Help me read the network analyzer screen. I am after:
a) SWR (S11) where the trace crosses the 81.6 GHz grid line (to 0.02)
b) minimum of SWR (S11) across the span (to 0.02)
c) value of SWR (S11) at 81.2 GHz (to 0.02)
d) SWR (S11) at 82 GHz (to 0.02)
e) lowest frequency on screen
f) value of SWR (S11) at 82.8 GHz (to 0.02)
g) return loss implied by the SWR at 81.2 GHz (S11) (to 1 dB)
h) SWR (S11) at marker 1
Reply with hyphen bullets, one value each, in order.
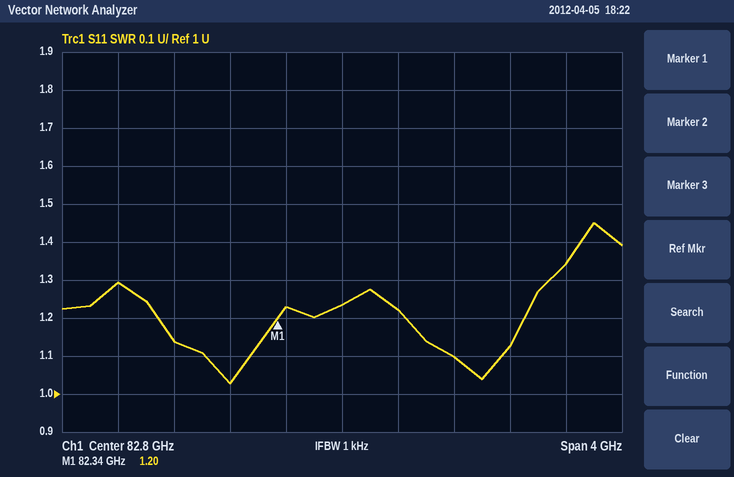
- 1.14
- 1.02
- 1.30
- 1.02
- 80.8 GHz
- 1.24
- 18 dB
- 1.20
